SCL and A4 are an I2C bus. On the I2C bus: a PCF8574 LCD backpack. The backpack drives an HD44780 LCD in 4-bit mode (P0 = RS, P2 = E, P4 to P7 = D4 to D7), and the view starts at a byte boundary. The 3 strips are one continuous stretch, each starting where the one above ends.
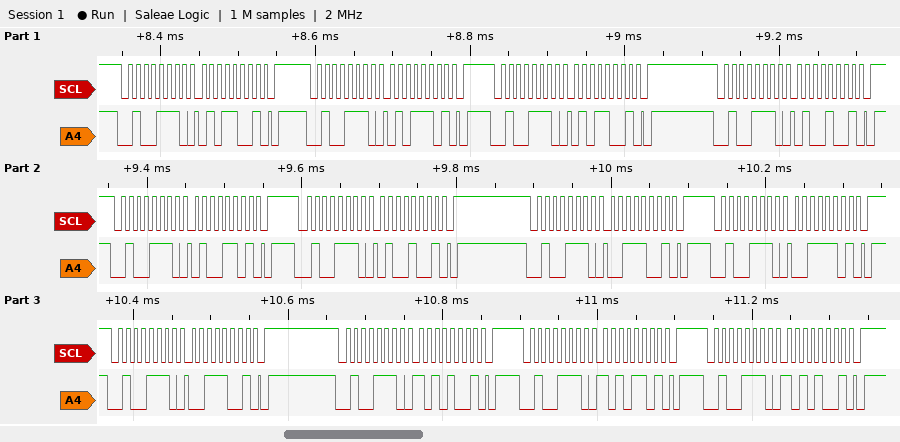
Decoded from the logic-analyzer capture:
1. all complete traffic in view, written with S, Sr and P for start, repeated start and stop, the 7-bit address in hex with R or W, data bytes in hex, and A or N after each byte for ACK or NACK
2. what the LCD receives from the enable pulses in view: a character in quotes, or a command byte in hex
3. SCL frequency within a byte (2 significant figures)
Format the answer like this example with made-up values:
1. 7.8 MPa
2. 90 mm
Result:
1. S 27W A 59 A P S 27W A 5D A P S 27W A 59 A P S 27W A 49 A P S 27W A 4D A P S 27W A 49 A P S 27W A 39 A P S 27W A 3D A P S 27W A 39 A P S 27W A A9 A P S 27W A AD A P S 27W A A9 A P
2. 'T' ':'
3. 100 kHz
